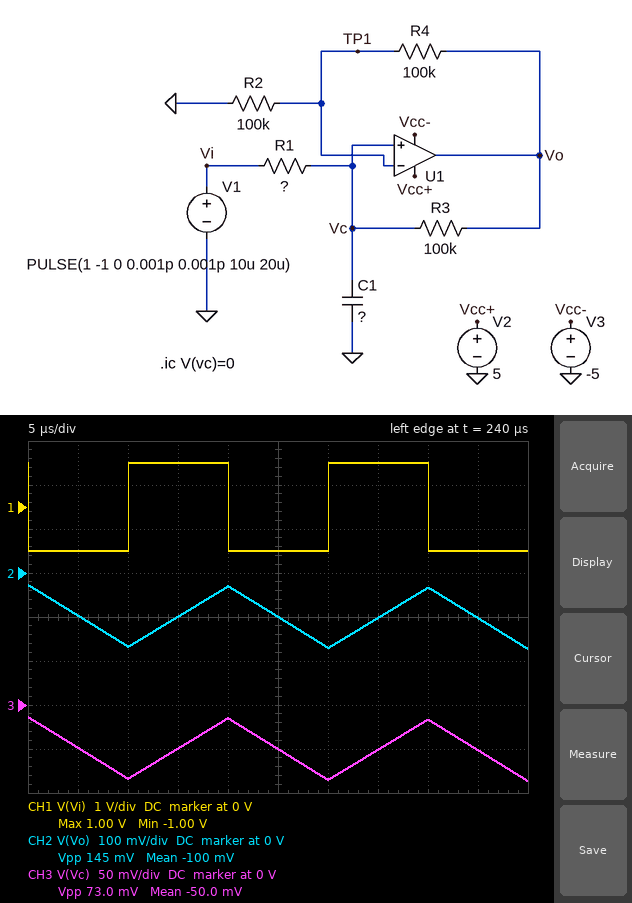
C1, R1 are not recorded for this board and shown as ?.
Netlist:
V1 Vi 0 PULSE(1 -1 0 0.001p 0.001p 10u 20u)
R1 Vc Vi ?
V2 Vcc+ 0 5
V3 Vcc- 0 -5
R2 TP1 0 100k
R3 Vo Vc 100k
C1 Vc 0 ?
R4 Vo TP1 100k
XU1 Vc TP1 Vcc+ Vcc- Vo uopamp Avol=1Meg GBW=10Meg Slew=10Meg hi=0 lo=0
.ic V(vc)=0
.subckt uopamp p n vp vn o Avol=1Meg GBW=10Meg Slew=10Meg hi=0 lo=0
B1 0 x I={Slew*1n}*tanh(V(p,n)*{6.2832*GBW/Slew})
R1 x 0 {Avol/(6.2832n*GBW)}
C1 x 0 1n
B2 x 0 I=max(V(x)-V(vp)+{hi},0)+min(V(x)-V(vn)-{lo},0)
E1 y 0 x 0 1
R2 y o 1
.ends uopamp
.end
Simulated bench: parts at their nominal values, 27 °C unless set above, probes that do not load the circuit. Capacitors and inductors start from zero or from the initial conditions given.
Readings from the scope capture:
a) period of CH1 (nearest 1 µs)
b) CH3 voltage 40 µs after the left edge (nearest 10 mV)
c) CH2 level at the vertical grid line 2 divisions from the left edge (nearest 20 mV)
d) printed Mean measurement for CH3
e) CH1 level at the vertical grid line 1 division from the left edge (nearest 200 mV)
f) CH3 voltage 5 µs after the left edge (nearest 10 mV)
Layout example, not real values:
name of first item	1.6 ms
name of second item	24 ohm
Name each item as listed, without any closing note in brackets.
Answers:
period of CH1	20 µs
CH3 voltage 40 µs after the left edge	-20 mV
CH2 level at the vertical grid line 2 divisions from the left edge	-160 mV
printed Mean measurement for CH3	-50.0 mV
CH1 level at the vertical grid line 1 division from the left edge	-1.0 V
CH3 voltage 5 µs after the left edge	-50 mV
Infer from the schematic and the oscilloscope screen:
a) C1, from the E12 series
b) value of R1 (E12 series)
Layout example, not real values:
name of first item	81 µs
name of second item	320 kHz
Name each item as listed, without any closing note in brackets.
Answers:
C1, from the E12 series	1.2 nF
value of R1	120 kΩ
